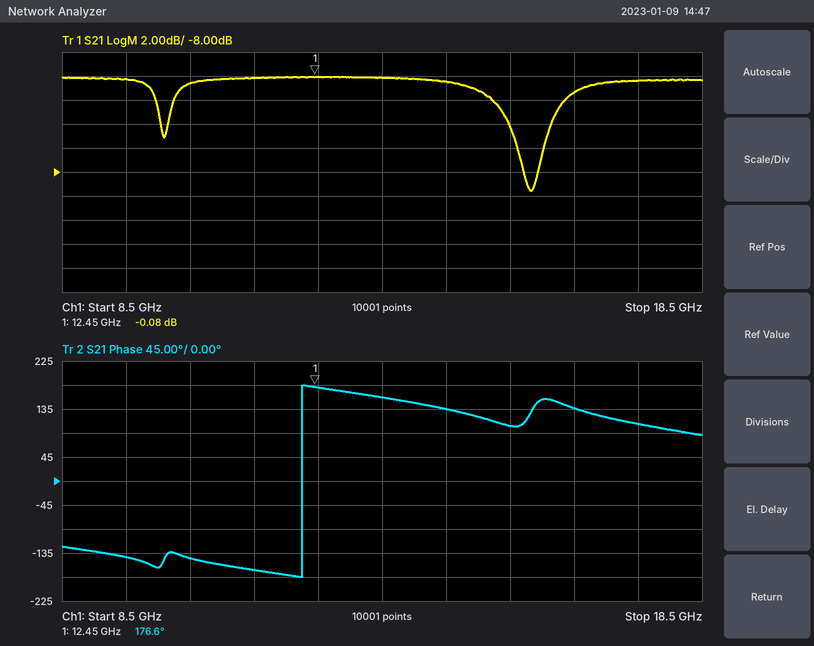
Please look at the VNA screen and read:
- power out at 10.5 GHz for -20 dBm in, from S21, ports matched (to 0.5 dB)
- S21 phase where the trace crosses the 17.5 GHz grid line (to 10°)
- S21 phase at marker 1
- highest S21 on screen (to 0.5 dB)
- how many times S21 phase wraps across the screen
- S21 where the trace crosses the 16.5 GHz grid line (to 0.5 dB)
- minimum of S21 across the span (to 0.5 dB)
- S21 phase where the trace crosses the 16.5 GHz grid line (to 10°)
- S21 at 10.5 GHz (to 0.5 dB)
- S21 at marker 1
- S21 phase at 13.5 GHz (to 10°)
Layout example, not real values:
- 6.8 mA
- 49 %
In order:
- -20.5 dBm
- 110°
- 176.6°
- 0.0 dB
- 1
- -1.5 dB
- -9.5 dB
- 140°
- -0.5 dB
- -0.08 dB
- 160°
